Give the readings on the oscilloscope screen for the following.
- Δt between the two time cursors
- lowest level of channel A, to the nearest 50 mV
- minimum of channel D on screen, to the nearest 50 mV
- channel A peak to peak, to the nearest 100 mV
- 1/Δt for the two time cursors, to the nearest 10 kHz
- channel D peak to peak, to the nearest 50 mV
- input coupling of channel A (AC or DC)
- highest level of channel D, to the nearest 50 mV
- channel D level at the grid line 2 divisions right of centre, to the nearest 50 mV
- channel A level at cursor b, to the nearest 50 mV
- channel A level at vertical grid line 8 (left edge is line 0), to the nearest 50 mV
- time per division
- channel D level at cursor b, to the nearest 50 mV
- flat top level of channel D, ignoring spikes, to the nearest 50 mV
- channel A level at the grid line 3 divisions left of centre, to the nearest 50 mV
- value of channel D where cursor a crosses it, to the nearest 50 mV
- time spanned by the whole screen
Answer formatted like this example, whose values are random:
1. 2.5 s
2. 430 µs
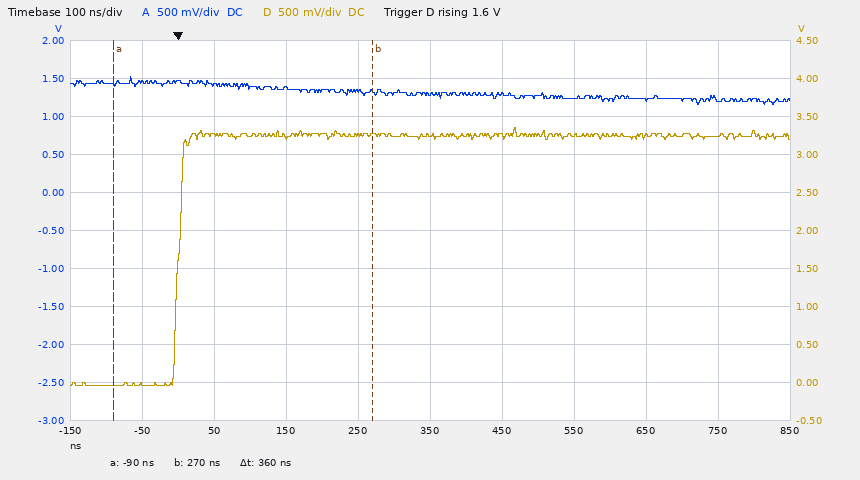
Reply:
1. 360 ns
2. 1.15 V
3. -50 mV
4. 400 mV
5. 2.78 MHz
6. 3.40 V
7. DC
8. 3.35 V
9. 3.25 V
10. 1.30 V
11. 1.20 V
12. 100 ns
13. 3.25 V
14. 3.25 V
15. 1.40 V
16. -50 mV
17. 1 µs
